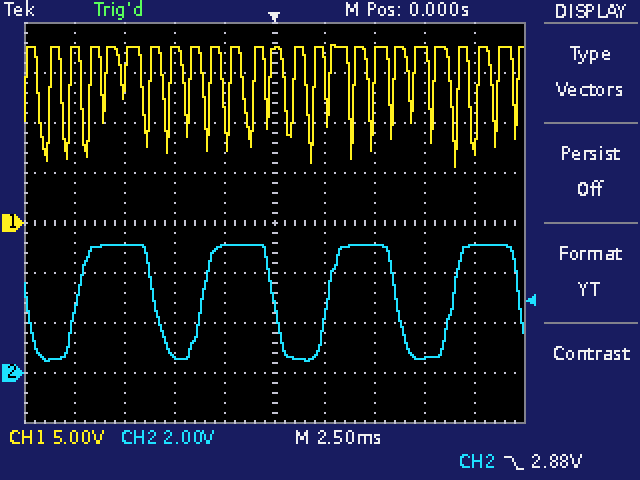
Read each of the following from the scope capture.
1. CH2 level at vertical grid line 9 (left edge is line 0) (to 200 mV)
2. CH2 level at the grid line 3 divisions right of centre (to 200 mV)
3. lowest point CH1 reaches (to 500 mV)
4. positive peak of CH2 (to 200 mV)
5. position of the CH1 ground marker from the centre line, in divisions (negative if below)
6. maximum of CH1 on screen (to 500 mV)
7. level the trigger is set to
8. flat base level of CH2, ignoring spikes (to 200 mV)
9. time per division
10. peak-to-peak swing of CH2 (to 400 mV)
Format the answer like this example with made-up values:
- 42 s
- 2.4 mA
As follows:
- 5.2 V
- 600 mV
- 5.5 V
- 5.2 V
- 0.0 div
- 18.0 V
- 2.88 V
- 600 mV
- 2.5 ms
- 4.8 V
